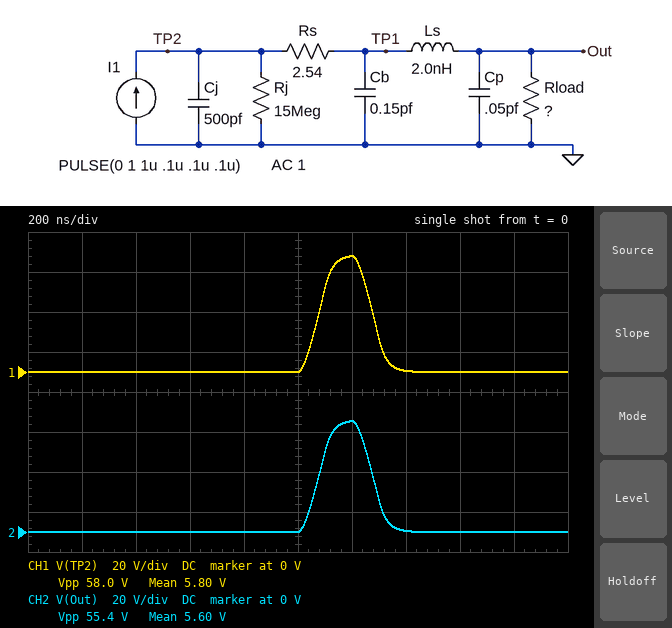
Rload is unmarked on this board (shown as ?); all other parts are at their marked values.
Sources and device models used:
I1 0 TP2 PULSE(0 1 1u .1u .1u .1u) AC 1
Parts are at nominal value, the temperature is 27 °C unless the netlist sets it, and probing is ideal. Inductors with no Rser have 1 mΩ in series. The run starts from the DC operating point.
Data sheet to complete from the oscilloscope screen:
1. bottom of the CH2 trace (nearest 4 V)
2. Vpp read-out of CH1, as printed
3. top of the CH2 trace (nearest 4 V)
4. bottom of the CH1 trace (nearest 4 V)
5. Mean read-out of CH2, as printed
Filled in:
0 V
58.0 V
56 V
0 V
5.60 V
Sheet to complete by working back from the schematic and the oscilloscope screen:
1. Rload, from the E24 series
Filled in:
56 Ω
